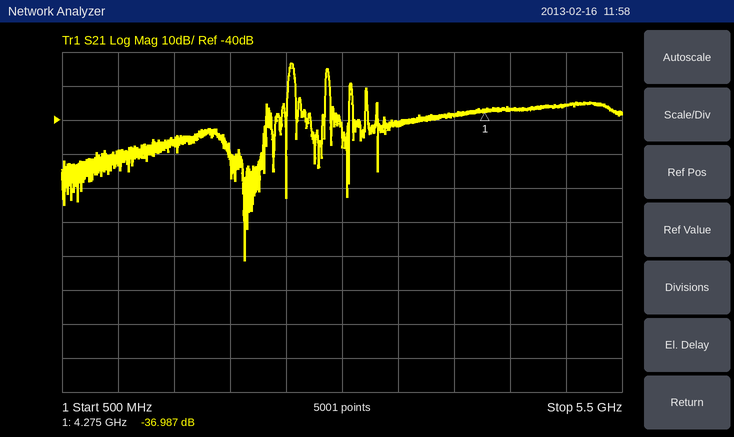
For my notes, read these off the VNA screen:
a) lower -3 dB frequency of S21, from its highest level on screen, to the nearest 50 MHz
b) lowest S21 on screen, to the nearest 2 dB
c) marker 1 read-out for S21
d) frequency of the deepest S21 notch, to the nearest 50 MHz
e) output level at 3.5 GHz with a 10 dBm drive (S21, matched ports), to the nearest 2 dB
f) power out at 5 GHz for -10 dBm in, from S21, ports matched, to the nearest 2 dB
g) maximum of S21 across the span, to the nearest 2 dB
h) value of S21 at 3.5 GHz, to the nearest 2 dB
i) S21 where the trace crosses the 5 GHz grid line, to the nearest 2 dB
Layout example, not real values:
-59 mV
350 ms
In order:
2.55 GHz
-82 dB
-36.987 dB
2.15 GHz
-32 dBm
-46 dBm
-24 dB
-42 dB
-36 dB
